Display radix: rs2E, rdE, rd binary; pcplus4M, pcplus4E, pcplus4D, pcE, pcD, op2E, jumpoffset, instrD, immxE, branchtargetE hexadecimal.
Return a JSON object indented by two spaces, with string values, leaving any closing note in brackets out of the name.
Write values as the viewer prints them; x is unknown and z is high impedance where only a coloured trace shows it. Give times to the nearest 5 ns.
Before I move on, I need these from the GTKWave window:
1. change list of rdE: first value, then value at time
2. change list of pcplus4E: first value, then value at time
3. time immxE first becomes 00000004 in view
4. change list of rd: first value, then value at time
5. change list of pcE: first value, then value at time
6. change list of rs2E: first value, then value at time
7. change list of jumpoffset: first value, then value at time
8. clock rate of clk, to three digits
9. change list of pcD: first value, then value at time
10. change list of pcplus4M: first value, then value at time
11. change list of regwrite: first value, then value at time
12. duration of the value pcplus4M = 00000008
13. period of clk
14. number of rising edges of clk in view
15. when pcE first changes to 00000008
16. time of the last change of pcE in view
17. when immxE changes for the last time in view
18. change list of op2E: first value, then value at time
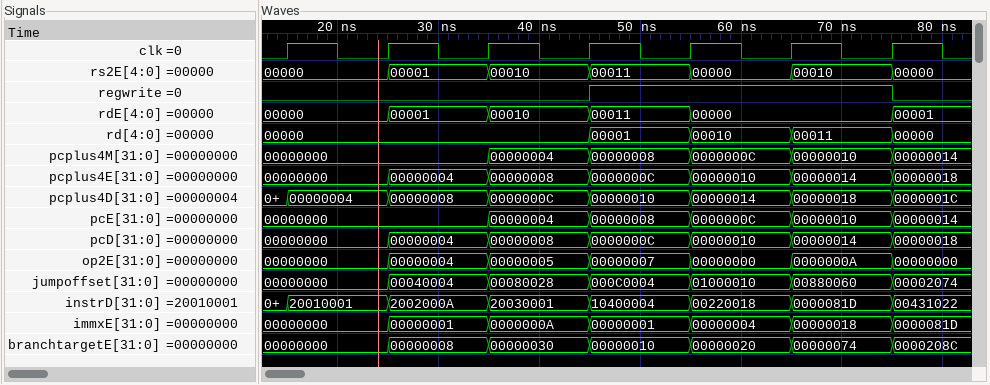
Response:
{
  "change list of rdE: first value, then value at time": "00000, 00001 at 25 ns, 00010 at 35 ns, 00011 at 45 ns, 00000 at 55 ns, 00001 at 75 ns",
  "change list of pcplus4E: first value, then value at time": "00000000, 00000004 at 25 ns, 00000008 at 35 ns, 0000000C at 45 ns, 00000010 at 55 ns, 00000014 at 65 ns, 00000018 at 75 ns",
  "time immxE first becomes 00000004 in view": "55 ns",
  "change list of rd: first value, then value at time": "00000, 00001 at 45 ns, 00010 at 55 ns, 00011 at 65 ns, 00000 at 75 ns",
  "change list of pcE: first value, then value at time": "00000000, 00000004 at 35 ns, 00000008 at 45 ns, 0000000C at 55 ns, 00000010 at 65 ns, 00000014 at 75 ns",
  "change list of rs2E: first value, then value at time": "00000, 00001 at 25 ns, 00010 at 35 ns, 00011 at 45 ns, 00000 at 55 ns, 00010 at 65 ns, 00000 at 75 ns",
  "change list of jumpoffset: first value, then value at time": "00000000, 00040004 at 25 ns, 00080028 at 35 ns, 000C0004 at 45 ns, 01000010 at 55 ns, 00880060 at 65 ns, 00002074 at 75 ns",
  "clock rate of clk, to three digits": "100 MHz",
  "change list of pcD: first value, then value at time": "00000000, 00000004 at 25 ns, 00000008 at 35 ns, 0000000C at 45 ns, 00000010 at 55 ns, 00000014 at 65 ns, 00000018 at 75 ns",
  "change list of pcplus4M: first value, then value at time": "00000000, 00000004 at 35 ns, 00000008 at 45 ns, 0000000C at 55 ns, 00000010 at 65 ns, 00000014 at 75 ns",
  "change list of regwrite: first value, then value at time": "0, 1 at 45 ns, 0 at 75 ns",
  "duration of the value pcplus4M = 00000008": "10 ns",
  "period of clk": "10 ns",
  "number of rising edges of clk in view": "7",
  "when pcE first changes to 00000008": "45 ns",
  "time of the last change of pcE in view": "75 ns",
  "when immxE changes for the last time in view": "75 ns",
  "change list of op2E: first value, then value at time": "00000000, 00000004 at 25 ns, 00000005 at 35 ns, 00000007 at 45 ns, 00000000 at 55 ns, 0000000A at 65 ns, 00000000 at 75 ns"
}
